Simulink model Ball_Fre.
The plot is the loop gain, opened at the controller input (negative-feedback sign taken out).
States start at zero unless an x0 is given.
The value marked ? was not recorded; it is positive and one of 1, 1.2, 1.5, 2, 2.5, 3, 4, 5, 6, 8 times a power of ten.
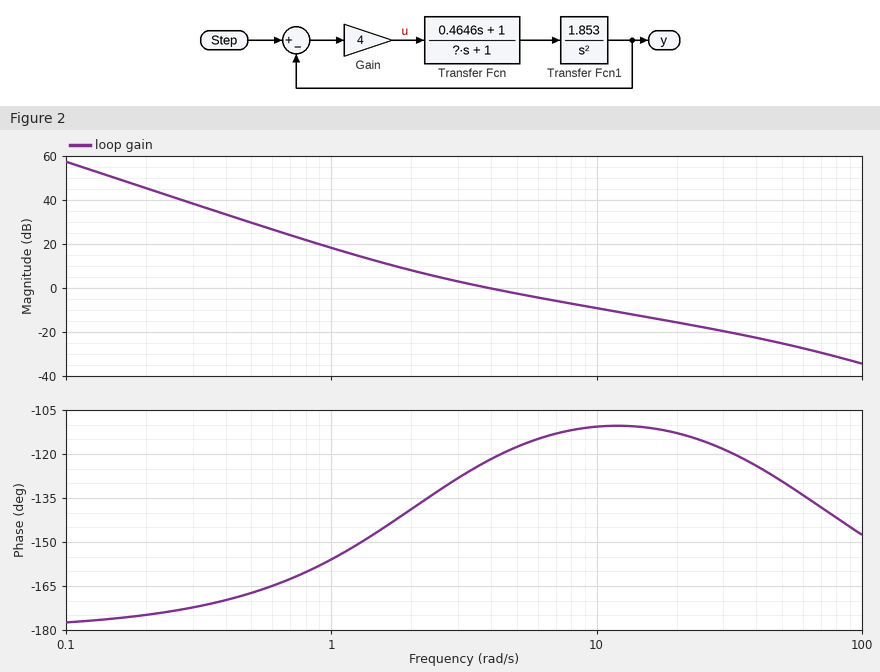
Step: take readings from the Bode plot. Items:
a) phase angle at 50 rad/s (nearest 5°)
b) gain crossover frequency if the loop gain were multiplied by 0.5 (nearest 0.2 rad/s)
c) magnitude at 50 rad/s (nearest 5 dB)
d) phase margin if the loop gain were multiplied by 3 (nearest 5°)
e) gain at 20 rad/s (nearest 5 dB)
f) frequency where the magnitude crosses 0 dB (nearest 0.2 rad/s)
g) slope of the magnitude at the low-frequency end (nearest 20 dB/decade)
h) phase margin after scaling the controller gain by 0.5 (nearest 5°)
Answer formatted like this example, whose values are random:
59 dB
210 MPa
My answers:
-130°
2.4 rad/s
-25 dB
70°
-15 dB
4.0 rad/s
-40 dB/decade
45°
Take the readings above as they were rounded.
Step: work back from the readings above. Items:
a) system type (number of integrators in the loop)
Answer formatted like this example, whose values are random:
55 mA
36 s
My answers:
2
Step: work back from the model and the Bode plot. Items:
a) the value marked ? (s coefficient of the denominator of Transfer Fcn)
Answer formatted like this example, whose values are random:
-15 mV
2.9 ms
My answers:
0.015
